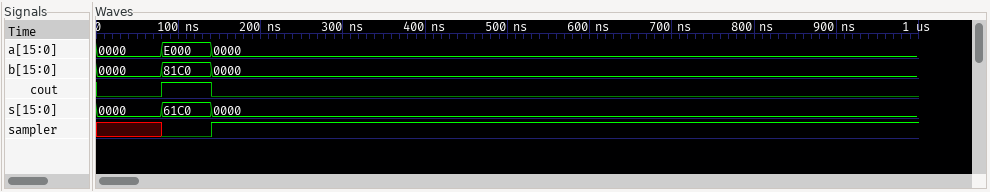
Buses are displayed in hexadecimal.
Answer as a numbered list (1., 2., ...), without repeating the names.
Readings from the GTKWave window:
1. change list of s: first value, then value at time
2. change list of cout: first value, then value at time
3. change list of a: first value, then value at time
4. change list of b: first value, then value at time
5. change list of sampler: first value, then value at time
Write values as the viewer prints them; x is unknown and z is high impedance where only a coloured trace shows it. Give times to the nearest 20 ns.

1. 0000, 61C0 at 80 ns, 0000 at 140 ns
2. 0, 1 at 80 ns, 0 at 140 ns
3. 0000, E000 at 80 ns, 0000 at 140 ns
4. 0000, 81C0 at 80 ns, 0000 at 140 ns
5. x, 0 at 80 ns, 1 at 140 ns
